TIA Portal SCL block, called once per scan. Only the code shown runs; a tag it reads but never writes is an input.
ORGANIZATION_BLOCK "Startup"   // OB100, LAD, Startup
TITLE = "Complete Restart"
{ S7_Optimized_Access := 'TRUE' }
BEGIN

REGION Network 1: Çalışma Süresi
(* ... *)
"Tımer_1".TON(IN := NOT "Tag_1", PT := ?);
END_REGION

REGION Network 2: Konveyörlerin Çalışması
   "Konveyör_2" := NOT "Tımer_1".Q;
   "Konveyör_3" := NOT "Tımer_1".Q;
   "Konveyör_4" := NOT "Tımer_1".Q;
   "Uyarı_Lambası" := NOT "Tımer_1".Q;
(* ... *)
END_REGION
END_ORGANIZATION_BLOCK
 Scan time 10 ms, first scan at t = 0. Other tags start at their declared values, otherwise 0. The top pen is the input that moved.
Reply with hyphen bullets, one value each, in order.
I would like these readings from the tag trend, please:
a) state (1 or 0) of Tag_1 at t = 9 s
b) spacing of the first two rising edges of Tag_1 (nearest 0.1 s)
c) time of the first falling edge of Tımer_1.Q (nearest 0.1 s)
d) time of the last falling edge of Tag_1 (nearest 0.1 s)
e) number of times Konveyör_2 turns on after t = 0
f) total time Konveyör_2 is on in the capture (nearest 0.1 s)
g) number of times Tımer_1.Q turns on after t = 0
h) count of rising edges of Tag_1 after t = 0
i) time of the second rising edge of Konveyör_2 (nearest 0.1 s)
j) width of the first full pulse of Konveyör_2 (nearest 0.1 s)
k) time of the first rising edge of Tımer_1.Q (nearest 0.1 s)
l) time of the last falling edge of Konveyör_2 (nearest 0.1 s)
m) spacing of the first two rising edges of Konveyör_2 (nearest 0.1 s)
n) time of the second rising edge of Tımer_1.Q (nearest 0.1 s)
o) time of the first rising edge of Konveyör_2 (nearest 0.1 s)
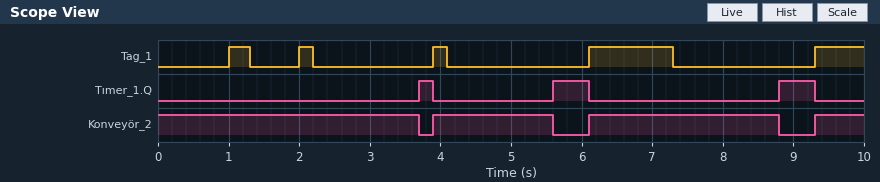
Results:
- 0
- 1.0 s
- 3.9 s
- 7.3 s
- 3
- 8.8 s
- 3
- 5
- 6.1 s
- 1.7 s
- 3.7 s
- 8.8 s
- 2.2 s
- 5.6 s
- 3.9 s
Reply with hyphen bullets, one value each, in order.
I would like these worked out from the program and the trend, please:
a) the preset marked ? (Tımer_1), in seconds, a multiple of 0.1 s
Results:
- 1.5 s
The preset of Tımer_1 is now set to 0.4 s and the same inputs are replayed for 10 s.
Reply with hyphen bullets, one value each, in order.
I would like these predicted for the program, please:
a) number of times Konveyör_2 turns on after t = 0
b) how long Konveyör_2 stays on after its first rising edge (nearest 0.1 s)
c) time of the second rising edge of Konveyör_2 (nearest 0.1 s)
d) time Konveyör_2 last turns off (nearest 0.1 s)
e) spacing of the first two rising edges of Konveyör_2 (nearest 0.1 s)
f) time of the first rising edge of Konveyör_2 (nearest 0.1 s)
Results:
- 5
- 0.7 s
- 2.0 s
- 7.7 s
- 1.0 s
- 1.0 s
